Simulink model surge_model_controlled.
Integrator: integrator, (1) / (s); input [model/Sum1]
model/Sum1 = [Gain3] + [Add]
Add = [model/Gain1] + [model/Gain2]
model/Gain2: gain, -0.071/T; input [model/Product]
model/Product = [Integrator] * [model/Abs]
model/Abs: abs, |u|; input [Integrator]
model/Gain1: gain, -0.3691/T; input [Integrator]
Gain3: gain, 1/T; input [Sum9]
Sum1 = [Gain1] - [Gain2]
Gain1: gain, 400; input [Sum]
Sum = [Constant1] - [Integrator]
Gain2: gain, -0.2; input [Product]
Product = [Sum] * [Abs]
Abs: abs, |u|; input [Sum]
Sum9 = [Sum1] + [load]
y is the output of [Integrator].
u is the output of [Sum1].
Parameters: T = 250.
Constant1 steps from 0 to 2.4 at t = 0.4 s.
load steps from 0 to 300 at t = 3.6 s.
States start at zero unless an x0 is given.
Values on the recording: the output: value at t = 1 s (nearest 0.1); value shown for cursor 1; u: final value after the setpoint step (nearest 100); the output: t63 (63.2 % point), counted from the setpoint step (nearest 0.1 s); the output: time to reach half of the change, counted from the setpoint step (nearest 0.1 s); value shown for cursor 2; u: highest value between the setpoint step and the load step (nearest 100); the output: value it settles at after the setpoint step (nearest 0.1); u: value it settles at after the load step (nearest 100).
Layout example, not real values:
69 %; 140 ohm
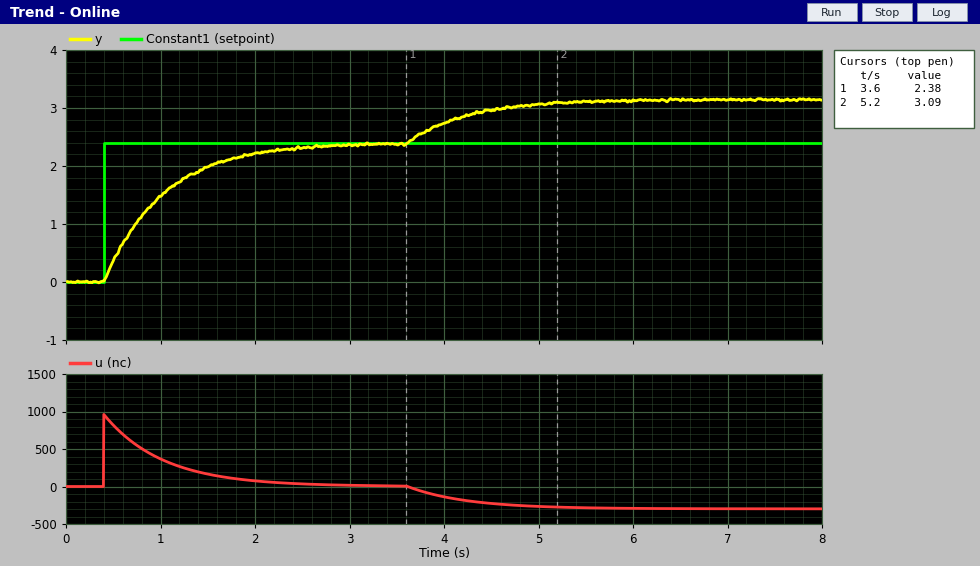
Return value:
1.5; 2.38; 0; 0.6 s; 0.4 s; 3.09; 1000; 2.4; -300
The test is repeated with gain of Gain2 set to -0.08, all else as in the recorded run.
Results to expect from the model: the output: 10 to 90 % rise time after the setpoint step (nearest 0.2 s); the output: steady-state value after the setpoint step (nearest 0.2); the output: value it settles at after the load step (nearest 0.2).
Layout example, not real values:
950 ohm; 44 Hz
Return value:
1.4 s; 2.4; 3.2
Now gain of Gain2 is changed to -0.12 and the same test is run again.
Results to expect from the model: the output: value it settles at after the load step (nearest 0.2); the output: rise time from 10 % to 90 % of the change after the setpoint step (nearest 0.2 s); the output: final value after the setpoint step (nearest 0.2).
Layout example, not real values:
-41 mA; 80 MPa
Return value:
3.2; 1.4 s; 2.4
